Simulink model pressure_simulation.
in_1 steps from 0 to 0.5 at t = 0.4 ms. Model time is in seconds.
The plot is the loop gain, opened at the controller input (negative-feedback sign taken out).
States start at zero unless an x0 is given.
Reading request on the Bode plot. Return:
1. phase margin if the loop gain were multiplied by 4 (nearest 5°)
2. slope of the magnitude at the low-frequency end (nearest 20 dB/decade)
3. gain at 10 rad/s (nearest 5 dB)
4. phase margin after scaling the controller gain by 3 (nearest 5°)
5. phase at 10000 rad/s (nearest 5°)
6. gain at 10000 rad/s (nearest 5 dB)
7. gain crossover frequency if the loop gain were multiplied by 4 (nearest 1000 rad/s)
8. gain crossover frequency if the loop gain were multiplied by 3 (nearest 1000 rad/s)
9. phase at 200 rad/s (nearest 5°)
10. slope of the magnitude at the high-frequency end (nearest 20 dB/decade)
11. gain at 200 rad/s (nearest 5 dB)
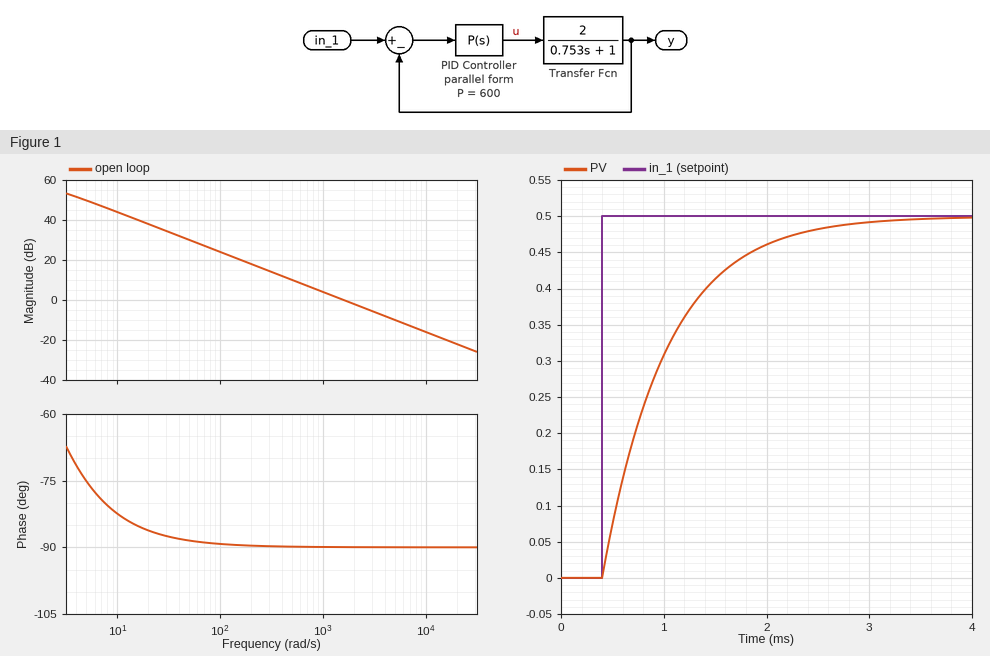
90°
-20 dB/decade
45 dB
90°
-90°
-15 dB
6000 rad/s
5000 rad/s
-90°
-20 dB/decade
20 dB
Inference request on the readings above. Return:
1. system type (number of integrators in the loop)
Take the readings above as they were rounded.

1
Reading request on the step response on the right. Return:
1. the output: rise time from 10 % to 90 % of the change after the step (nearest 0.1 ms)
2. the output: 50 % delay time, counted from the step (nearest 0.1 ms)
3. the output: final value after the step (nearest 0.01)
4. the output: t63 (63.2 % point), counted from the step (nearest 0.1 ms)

1.4 ms
0.4 ms
0.50
0.6 ms
